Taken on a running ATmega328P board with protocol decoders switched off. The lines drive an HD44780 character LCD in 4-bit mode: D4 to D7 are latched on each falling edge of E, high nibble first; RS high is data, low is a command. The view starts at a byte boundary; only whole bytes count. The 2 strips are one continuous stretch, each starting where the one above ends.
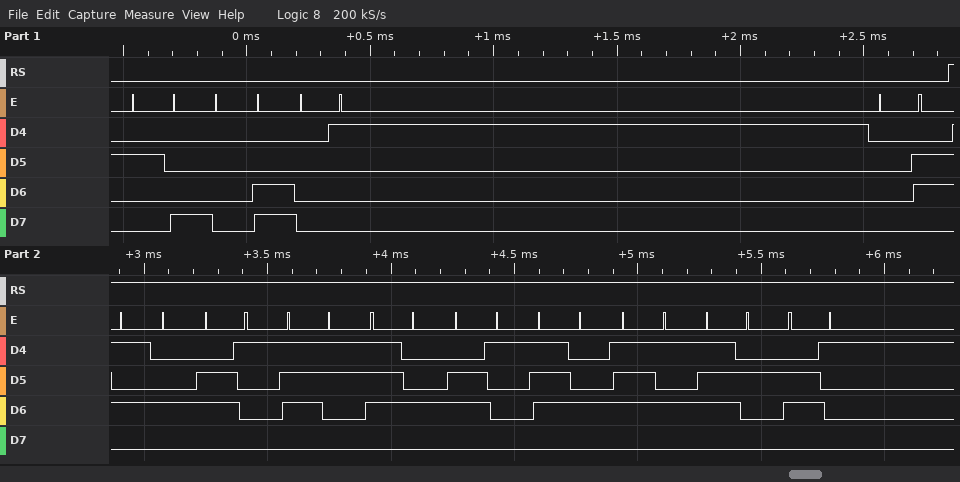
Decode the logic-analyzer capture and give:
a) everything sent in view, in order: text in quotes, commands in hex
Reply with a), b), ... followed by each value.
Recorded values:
a) 0x28 0x0C 0x01 0x06 "Tastatura"
